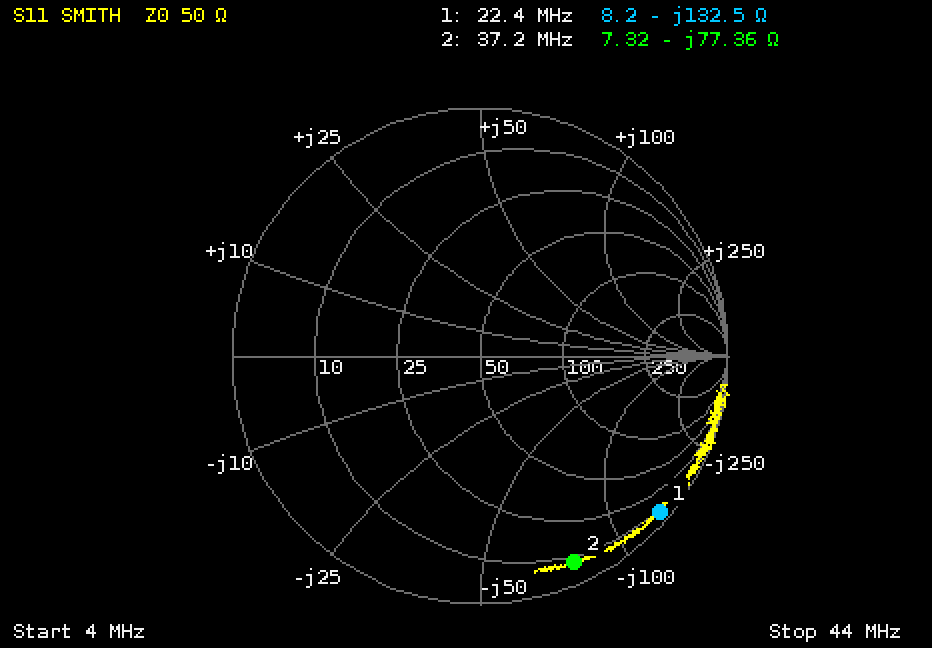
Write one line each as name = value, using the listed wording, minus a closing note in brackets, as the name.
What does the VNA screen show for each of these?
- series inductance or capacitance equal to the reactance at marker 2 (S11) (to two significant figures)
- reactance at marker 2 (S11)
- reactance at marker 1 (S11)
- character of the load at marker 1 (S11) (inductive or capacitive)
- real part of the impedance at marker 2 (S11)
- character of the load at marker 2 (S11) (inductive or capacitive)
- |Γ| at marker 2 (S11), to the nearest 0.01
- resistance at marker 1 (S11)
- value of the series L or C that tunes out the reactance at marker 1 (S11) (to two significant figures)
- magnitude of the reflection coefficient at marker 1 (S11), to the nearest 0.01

series inductance or capacitance equal to the reactance at marker 2 (S11) = 55 pF
reactance at marker 2 = -77.36 Ω
reactance at marker 1 = -132.5 Ω
character of the load at marker 1 (S11) = capacitive
real part of the impedance at marker 2 = 7.32 Ω
character of the load at marker 2 (S11) = capacitive
|Γ| at marker 2 (S11), to the nearest 0.01 = 0.92
resistance at marker 1 = 8.2 Ω
value of the series L or C that tunes out the reactance at marker 1 (S11) = 940 nH
magnitude of the reflection coefficient at marker 1 (S11), to the nearest 0.01 = 0.96
